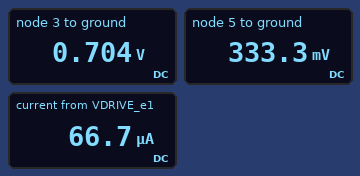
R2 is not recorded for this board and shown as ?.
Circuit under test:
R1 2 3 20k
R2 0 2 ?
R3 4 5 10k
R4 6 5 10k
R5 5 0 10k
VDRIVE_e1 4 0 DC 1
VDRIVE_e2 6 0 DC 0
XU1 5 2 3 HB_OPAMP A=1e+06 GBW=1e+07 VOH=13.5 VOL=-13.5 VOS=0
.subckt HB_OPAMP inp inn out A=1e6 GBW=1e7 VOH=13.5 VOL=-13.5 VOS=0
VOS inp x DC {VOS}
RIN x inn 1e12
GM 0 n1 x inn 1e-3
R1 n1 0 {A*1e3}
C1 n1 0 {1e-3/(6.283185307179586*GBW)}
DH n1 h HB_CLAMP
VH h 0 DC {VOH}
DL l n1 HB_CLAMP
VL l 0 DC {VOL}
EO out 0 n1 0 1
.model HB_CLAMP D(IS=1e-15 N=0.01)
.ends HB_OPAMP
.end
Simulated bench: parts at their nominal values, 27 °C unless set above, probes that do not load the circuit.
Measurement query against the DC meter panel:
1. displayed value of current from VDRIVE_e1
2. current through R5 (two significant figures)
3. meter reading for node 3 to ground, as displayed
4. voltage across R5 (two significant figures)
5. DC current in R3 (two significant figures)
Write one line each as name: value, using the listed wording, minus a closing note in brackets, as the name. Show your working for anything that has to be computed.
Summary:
displayed value of current from VDRIVE_e1: 66.7 µA
current through R5: (333.3 mV) / 10 kΩ = 33 µA
meter reading for node 3 to ground, as displayed: 0.704 V
voltage across R5: 333.3 mV = 330 mV
DC current in R3: (1 V - 333.3 mV) / 10 kΩ = 67 µA
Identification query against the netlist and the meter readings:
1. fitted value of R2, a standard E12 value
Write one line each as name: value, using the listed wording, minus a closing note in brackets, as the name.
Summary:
fitted value of R2, a standard E12 value: 18 kΩ
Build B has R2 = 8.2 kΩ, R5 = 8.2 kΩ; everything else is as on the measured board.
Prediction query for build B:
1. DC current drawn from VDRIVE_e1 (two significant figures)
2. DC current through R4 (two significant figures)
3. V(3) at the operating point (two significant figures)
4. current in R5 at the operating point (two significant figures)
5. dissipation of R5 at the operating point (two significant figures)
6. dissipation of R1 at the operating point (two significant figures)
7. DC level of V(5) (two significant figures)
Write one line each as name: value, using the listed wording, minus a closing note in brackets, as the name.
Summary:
DC current drawn from VDRIVE_e1: 69 µA
DC current through R4: 31 µA
V(3) at the operating point: 1.1 V
current in R5 at the operating point: 38 µA
dissipation of R5 at the operating point: 12 µW
dissipation of R1 at the operating point: 29 µW
DC level of V(5): 310 mV
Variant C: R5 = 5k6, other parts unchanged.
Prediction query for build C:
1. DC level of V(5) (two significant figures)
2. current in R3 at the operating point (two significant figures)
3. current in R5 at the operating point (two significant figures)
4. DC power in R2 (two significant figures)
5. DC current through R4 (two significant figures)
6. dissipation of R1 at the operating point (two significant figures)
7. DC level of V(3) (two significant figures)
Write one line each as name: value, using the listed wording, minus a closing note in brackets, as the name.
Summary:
DC level of V(5): 260 mV
current in R3 at the operating point: 74 µA
current in R5 at the operating point: 47 µA
DC power in R2: 3.9 µW
DC current through R4: 26 µA
dissipation of R1 at the operating point: 4.3 µW
DC level of V(3): 560 mV
